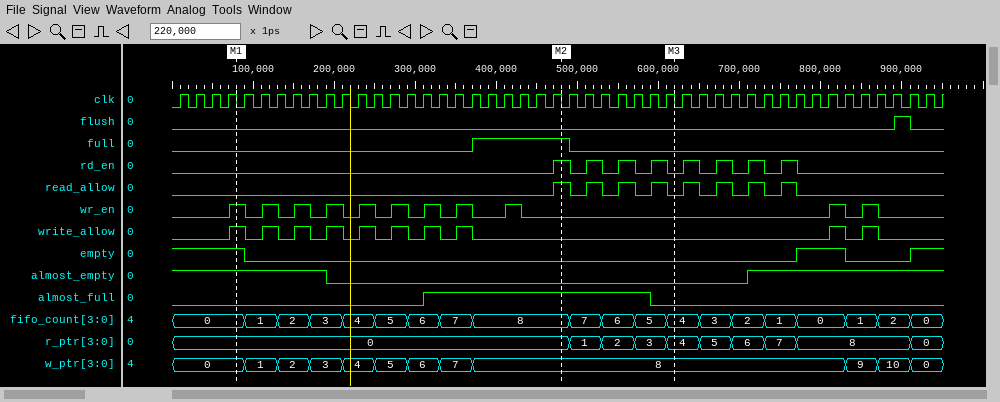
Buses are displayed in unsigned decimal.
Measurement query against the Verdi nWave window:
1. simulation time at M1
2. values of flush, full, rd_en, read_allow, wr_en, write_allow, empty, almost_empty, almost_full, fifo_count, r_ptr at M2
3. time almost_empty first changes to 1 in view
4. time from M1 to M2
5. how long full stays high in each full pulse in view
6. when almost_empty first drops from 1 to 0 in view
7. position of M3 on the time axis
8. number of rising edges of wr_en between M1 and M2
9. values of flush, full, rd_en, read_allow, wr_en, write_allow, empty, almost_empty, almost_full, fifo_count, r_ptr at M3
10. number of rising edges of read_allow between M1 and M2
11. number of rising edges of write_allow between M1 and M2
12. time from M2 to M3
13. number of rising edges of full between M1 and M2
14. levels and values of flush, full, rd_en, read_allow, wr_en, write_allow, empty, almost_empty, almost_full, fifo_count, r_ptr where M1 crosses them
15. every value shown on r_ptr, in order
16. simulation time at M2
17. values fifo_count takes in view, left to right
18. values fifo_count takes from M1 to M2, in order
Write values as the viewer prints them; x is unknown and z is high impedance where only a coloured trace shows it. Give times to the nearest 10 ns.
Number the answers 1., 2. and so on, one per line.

1. 80 ns
2. flush=0, full=1, rd_en=1, read_allow=1, wr_en=0, write_allow=0, empty=0, almost_empty=0, almost_full=1, fifo_count=8, r_ptr=0
3. 710 ns
4. 400 ns
5. 120 ns
6. 190 ns
7. 620 ns
8. 8
9. flush=0, full=0, rd_en=0, read_allow=0, wr_en=0, write_allow=0, empty=0, almost_empty=0, almost_full=0, fifo_count=4, r_ptr=4
10. 1
11. 7
12. 140 ns
13. 1
14. flush=0, full=0, rd_en=0, read_allow=0, wr_en=1, write_allow=1, empty=1, almost_empty=1, almost_full=0, fifo_count=0, r_ptr=0
15. 0, 1, 2, 3, 4, 5, 6, 7, 8, 0
16. 480 ns
17. 0, 1, 2, 3, 4, 5, 6, 7, 8, 7, 6, 5, 4, 3, 2, 1, 0, 1, 2, 0
18. 0, 1, 2, 3, 4, 5, 6, 7, 8
